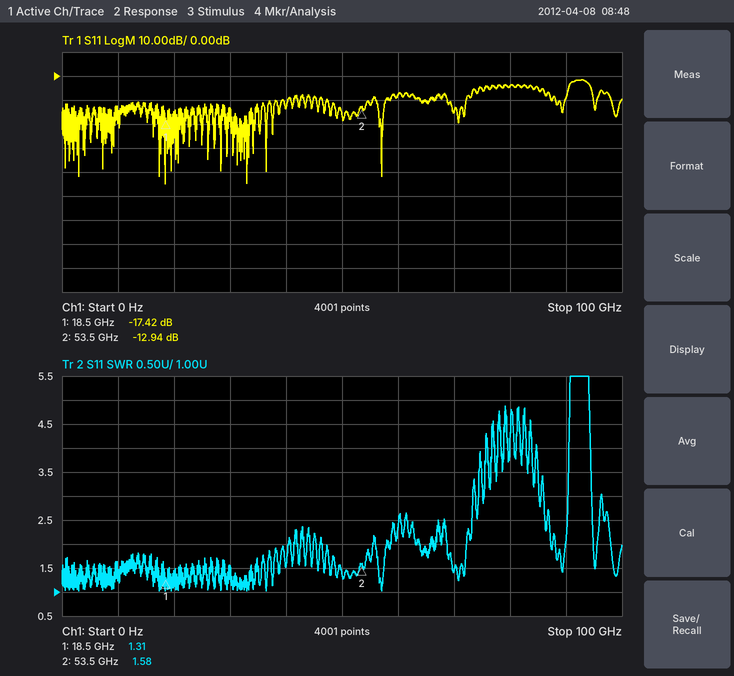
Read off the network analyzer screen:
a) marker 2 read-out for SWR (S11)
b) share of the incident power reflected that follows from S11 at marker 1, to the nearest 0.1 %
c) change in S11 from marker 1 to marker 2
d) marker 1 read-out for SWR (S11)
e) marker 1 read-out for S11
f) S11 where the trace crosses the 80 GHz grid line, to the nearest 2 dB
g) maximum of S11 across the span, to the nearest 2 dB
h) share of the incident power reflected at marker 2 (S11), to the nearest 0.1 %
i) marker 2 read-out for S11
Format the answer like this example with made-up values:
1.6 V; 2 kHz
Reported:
1.58; 1.8 %; 4.48 dB; 1.31; -17.42 dB; -4 dB; -2 dB; 5.1 %; -12.94 dB
